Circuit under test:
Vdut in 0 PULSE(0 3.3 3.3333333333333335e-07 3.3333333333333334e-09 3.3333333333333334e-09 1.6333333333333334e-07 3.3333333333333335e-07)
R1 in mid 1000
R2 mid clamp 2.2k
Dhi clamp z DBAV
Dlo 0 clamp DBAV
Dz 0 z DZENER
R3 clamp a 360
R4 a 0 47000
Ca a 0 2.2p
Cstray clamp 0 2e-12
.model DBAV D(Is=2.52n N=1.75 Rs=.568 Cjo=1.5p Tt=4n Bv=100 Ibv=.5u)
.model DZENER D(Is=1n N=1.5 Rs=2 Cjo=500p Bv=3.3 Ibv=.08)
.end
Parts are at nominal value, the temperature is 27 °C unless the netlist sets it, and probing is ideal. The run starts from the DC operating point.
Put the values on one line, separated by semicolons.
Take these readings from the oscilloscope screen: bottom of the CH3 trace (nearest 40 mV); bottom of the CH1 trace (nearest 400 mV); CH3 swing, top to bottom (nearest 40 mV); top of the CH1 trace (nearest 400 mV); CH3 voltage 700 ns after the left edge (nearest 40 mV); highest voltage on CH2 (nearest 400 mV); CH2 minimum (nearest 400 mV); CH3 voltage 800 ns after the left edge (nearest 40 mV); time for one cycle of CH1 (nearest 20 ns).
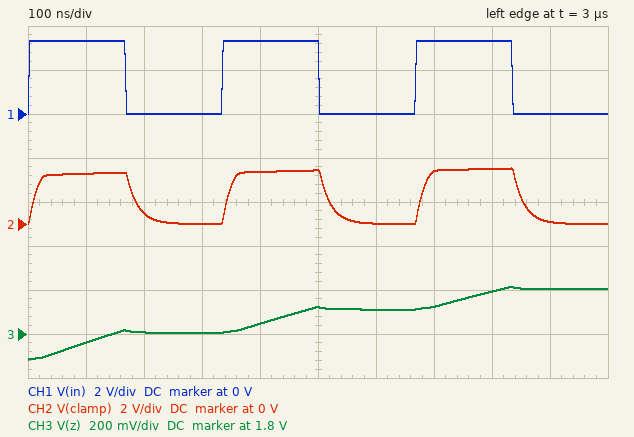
1.68 V; 0 V; 320 mV; 3.2 V; 1.92 V; 2.4 V; 0 V; 2.00 V; 340 ns
